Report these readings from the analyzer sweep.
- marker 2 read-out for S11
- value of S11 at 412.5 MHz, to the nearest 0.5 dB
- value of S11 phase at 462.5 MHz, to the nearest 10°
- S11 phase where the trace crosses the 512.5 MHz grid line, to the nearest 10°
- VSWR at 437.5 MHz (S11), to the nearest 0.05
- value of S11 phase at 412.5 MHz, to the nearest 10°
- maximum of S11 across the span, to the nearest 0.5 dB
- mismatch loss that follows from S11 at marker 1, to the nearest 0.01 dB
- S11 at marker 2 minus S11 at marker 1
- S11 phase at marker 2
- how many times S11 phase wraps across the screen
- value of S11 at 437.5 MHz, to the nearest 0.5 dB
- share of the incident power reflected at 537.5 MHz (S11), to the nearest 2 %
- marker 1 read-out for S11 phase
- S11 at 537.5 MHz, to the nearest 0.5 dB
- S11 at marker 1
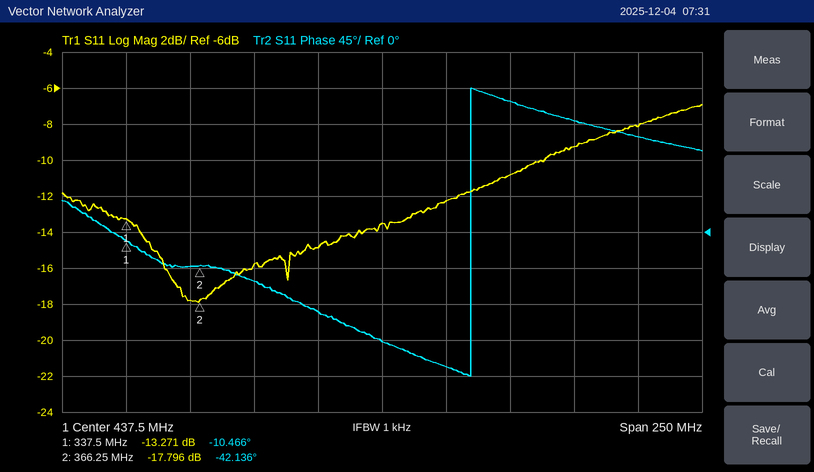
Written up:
-17.796 dB
-15.0 dB
-170°
140°
1.55
-100°
-7.0 dB
0.21 dB
-4.525 dB
-42.136°
1
-13.5 dB
16 %
-10.466°
-8.0 dB
-13.271 dB
